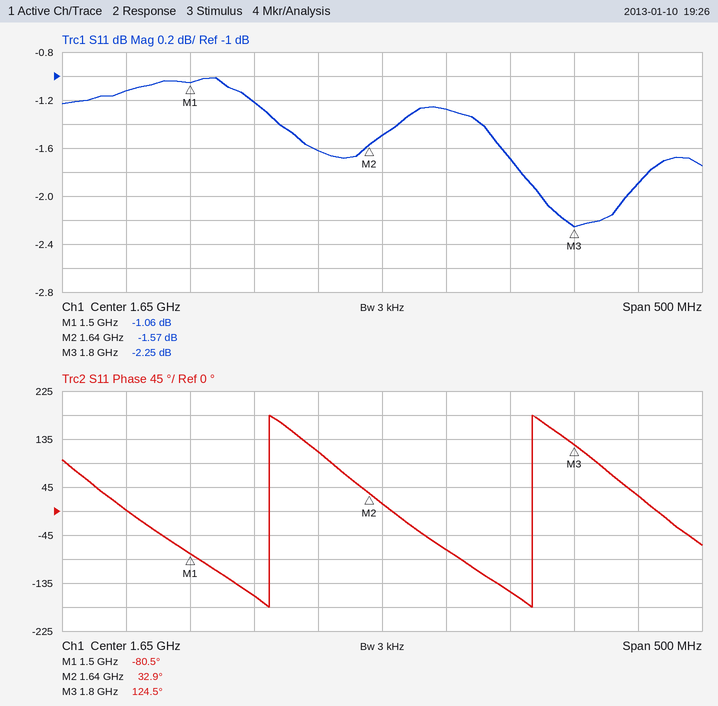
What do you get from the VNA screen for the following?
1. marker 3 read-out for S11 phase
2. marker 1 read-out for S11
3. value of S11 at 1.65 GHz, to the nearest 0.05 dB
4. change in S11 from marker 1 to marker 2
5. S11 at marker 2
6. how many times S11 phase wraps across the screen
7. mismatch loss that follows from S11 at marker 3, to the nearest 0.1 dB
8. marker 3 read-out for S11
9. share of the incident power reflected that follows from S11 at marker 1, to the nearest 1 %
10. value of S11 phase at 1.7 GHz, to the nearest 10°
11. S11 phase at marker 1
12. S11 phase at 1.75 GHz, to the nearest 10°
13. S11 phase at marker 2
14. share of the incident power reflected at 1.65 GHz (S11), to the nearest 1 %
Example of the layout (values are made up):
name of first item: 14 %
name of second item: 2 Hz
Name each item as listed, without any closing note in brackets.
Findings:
marker 3 read-out for S11 phase: 124.5°
marker 1 read-out for S11: -1.06 dB
value of S11 at 1.65 GHz, to the nearest 0.05 dB: -1.50 dB
change in S11 from marker 1 to marker 2: -0.51 dB
S11 at marker 2: -1.57 dB
how many times S11 phase wraps across the screen: 2
mismatch loss that follows from S11 at marker 3, to the nearest 0.1 dB: 3.9 dB
marker 3 read-out for S11: -2.25 dB
share of the incident power reflected that follows from S11 at marker 1, to the nearest 1 %: 78 %
value of S11 phase at 1.7 GHz, to the nearest 10°: -70°
S11 phase at marker 1: -80.5°
S11 phase at 1.75 GHz, to the nearest 10°: -150°
S11 phase at marker 2: 32.9°
share of the incident power reflected at 1.65 GHz (S11), to the nearest 1 %: 71 %
